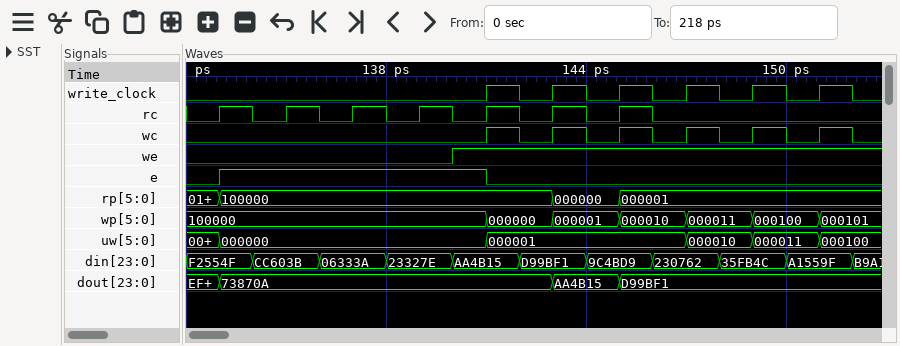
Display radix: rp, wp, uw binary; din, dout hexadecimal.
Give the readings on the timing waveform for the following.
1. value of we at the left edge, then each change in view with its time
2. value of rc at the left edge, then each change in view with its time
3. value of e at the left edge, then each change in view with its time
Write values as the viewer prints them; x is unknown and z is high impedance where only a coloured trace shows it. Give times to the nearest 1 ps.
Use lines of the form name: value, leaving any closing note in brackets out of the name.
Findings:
value of we at the left edge, then each change in view with its time: 0, 1 at 140 ps
value of rc at the left edge, then each change in view with its time: 0, 1 at 133 ps, 0 at 134 ps, 1 at 135 ps, 0 at 136 ps, 1 at 137 ps, 0 at 138 ps, 1 at 139 ps, 0 at 140 ps, 1 at 141 ps, 0 at 142 ps, 1 at 143 ps, 0 at 144 ps, 1 at 145 ps, 0 at 146 ps
value of e at the left edge, then each change in view with its time: 0, 1 at 133 ps, 0 at 141 ps
